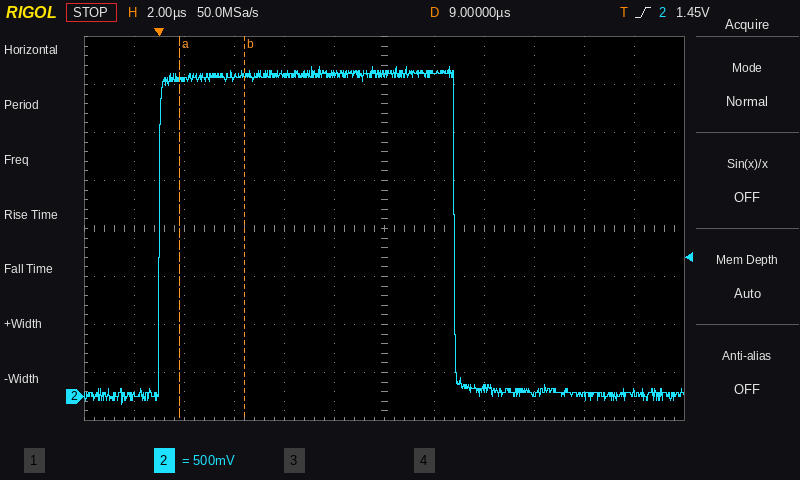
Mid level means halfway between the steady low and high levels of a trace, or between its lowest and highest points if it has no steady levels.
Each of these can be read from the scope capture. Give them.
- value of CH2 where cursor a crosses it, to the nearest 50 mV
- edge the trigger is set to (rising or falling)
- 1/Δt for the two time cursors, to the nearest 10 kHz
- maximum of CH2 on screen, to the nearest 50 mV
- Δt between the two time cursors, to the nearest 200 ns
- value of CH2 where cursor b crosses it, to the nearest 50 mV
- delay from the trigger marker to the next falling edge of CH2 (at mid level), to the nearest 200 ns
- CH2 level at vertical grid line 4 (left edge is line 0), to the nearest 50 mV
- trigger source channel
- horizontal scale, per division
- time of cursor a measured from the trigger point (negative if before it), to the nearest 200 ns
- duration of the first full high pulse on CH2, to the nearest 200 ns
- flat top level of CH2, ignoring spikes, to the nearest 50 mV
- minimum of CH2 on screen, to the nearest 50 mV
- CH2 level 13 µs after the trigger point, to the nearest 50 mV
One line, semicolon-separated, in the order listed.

3.30 V; rising; 380 kHz; 3.45 V; 2.6 µs; 3.35 V; 11.8 µs; 3.35 V; CH2; 2 µs; +800 ns; 11.8 µs; 3.35 V; -100 mV; 100 mV
